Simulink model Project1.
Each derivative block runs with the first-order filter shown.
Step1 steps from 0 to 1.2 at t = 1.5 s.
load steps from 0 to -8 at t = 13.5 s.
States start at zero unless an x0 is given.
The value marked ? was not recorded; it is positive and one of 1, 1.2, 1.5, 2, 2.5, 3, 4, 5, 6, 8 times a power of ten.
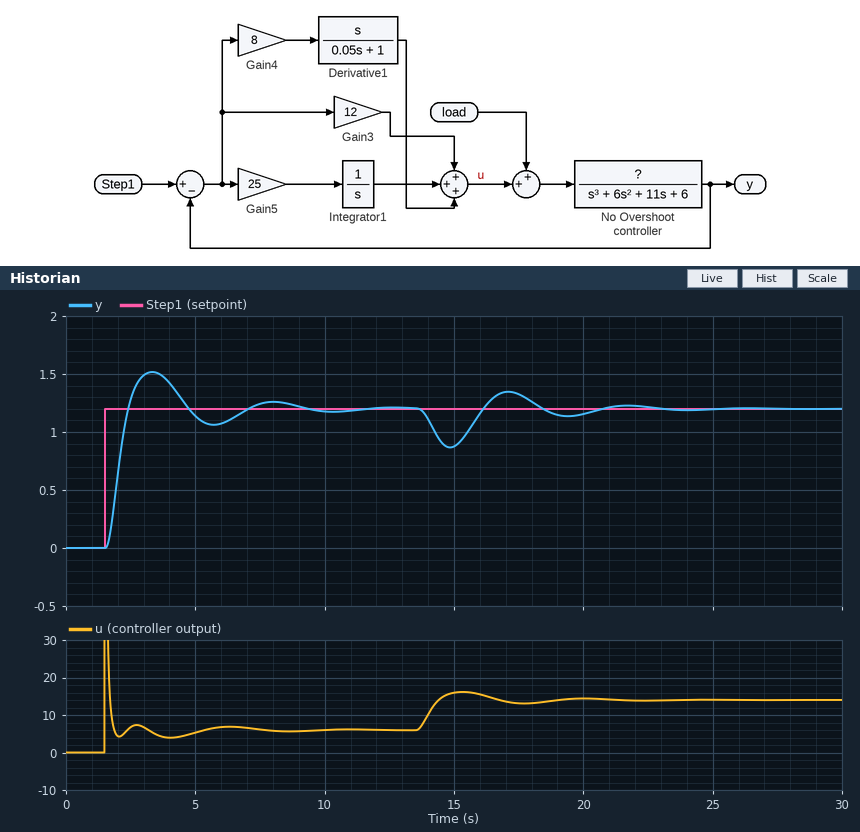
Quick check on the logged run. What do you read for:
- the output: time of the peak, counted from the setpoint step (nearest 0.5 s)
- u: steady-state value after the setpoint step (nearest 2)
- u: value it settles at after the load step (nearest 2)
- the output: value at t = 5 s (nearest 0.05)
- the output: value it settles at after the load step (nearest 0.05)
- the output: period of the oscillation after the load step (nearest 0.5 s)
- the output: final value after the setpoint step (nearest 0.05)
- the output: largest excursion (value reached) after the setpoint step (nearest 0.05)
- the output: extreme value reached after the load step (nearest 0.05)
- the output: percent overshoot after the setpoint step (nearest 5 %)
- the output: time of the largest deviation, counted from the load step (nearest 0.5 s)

2.0 s
6
14
1.15
1.20
4.5 s
1.20
1.50
0.85
25 %
1.5 s
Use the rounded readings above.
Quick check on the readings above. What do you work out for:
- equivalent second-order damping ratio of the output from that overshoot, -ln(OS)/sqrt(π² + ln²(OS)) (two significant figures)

0.40
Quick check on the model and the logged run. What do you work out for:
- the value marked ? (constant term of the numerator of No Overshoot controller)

1.2
